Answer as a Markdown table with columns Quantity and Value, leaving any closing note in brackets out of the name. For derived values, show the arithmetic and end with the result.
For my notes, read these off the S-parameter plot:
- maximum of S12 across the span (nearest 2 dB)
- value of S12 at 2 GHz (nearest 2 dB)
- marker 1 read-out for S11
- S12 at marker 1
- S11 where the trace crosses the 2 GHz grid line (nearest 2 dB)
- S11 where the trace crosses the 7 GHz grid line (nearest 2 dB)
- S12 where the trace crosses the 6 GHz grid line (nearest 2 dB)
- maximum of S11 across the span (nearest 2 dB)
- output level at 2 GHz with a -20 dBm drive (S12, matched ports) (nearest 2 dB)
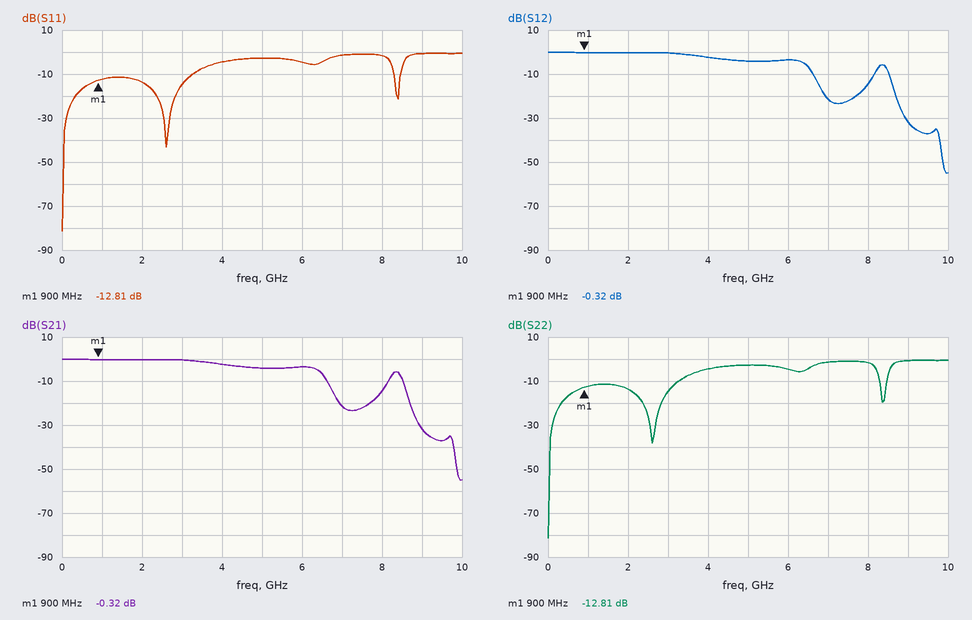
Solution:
| Quantity | Value |
|---|---|
| maximum of S12 across the span | 0 dB |
| value of S12 at 2 GHz | 0 dB |
| marker 1 read-out for S11 | -12.81 dB |
| S12 at marker 1 | -0.32 dB |
| S11 where the trace crosses the 2 GHz grid line | -14 dB |
| S11 where the trace crosses the 7 GHz grid line | -2 dB |
| S12 where the trace crosses the 6 GHz grid line | -4 dB |
| maximum of S11 across the span | 0 dB |
| output level at 2 GHz with a -20 dBm drive (S12, matched ports) | -20 dBm + (0 dB) = -20 dBm |
